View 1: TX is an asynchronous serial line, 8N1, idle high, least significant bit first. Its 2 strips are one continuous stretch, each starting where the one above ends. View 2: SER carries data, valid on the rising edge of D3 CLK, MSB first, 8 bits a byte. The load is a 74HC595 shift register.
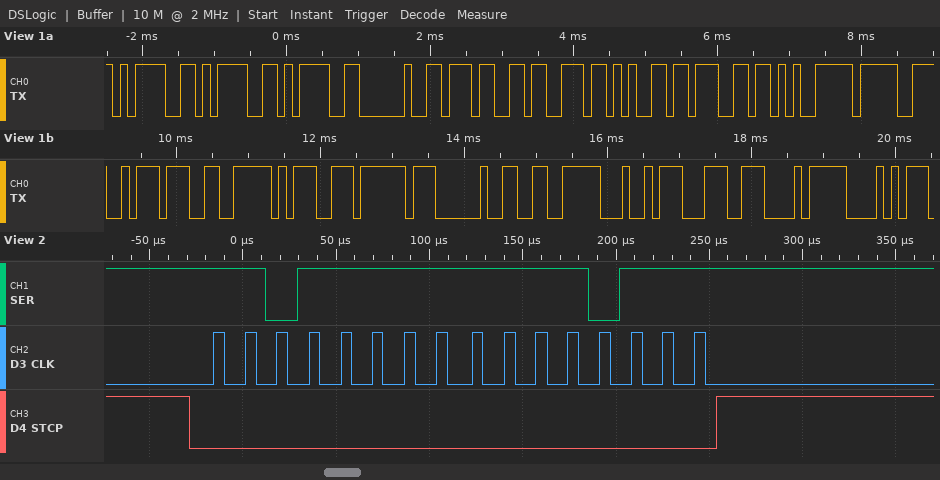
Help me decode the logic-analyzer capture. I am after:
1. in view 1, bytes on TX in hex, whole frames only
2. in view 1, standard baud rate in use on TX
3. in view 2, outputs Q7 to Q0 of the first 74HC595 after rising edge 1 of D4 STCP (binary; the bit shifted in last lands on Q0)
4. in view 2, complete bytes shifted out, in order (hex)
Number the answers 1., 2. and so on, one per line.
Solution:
1. 3D 3D 3D 20 37 73 65 67 E5 9F BA E6 9D BF 20 E6 A4 9C E8 A8
2. 9600 baud
3. 11110111
4. 0xDF 0xF7
